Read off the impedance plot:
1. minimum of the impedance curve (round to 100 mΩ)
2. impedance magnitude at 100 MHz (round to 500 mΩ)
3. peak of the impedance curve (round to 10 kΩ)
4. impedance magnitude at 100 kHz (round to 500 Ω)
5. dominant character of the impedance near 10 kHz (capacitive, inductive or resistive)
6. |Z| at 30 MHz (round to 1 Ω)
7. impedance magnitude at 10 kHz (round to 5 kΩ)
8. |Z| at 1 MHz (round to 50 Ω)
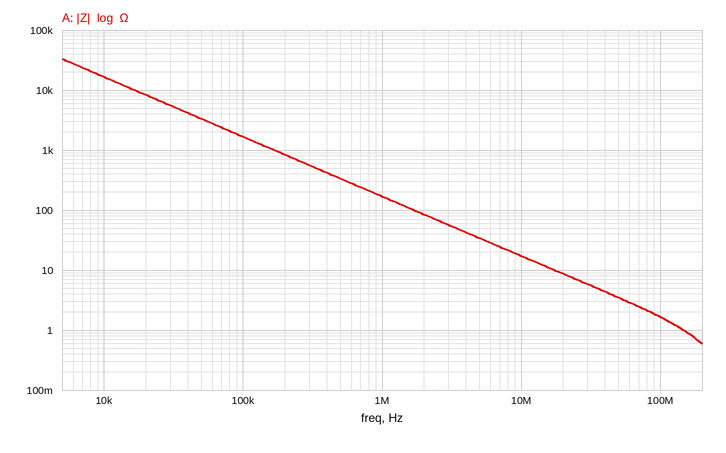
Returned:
600 mΩ
1.5 Ω
30 kΩ
1.5 kΩ
capacitive
6 Ω
15 kΩ
150 Ω
